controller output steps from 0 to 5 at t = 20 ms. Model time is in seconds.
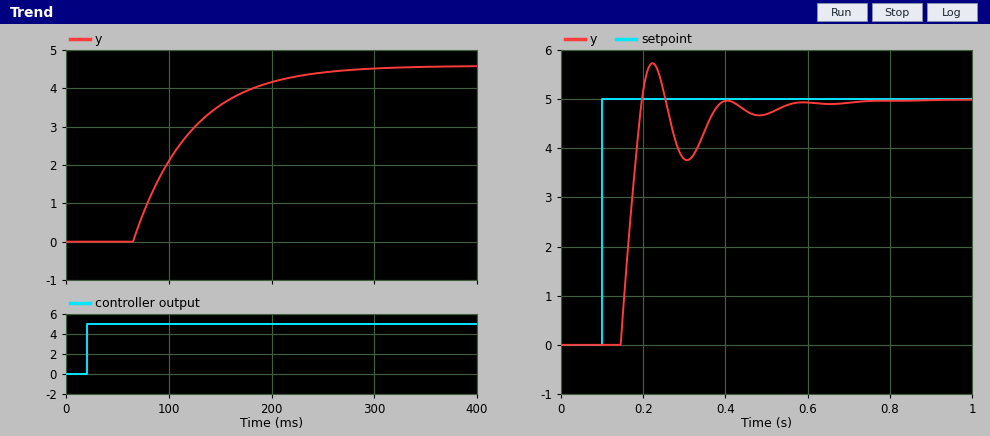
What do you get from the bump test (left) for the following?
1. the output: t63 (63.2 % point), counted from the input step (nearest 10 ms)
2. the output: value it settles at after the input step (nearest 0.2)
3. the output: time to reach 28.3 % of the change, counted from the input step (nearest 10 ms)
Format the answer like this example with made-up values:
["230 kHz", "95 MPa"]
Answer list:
["100 ms", "4.6", "60 ms"]
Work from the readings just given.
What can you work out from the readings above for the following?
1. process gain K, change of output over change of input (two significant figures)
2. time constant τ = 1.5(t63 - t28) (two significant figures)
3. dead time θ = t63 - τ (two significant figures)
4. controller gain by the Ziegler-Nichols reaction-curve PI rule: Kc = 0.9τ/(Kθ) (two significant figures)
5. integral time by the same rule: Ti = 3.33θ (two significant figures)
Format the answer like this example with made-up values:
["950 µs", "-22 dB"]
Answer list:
["0.92", "60 ms", "40 ms", "1.5", "130 ms"]
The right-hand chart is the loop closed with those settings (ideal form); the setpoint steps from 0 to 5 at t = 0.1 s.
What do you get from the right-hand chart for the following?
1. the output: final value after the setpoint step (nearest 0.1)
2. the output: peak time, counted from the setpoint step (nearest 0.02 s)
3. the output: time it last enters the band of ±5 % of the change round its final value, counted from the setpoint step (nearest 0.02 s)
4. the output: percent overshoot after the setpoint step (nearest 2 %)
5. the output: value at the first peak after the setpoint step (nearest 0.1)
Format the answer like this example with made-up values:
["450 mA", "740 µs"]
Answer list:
["5.0", "0.12 s", "0.42 s", "14 %", "5.7"]
